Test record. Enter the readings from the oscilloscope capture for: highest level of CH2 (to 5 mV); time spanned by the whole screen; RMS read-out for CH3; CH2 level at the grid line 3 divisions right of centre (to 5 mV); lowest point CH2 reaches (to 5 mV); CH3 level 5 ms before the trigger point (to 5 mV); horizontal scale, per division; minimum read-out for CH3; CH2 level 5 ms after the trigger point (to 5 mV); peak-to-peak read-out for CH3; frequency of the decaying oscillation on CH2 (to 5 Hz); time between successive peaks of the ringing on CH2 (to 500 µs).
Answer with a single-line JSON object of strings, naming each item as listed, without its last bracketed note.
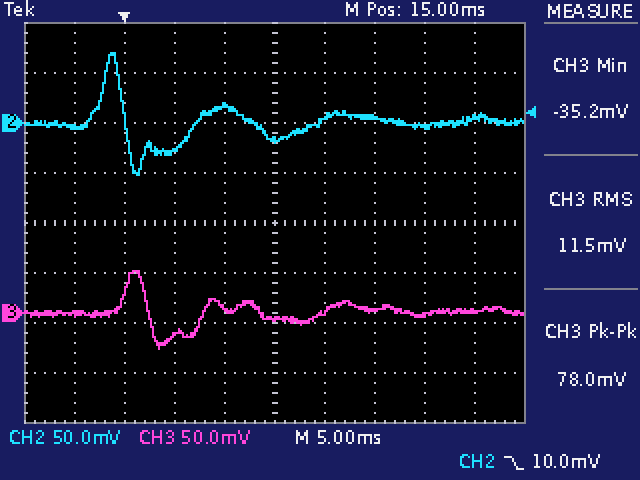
{"highest level of CH2": "70 mV", "time spanned by the whole screen": "50 ms", "RMS read-out for CH3": "11.5 mV", "CH2 level at the grid line 3 divisions right of centre": "-5 mV", "lowest point CH2 reaches": "-50 mV", "CH3 level 5 ms before the trigger point": "0 mV", "horizontal scale, per division": "5 ms", "minimum read-out for CH3": "-35.2 mV", "CH2 level 5 ms after the trigger point": "-30 mV", "peak-to-peak read-out for CH3": "78.0 mV", "frequency of the decaying oscillation on CH2": "90 Hz", "time between successive peaks of the ringing on CH2": "11.0 ms"}
